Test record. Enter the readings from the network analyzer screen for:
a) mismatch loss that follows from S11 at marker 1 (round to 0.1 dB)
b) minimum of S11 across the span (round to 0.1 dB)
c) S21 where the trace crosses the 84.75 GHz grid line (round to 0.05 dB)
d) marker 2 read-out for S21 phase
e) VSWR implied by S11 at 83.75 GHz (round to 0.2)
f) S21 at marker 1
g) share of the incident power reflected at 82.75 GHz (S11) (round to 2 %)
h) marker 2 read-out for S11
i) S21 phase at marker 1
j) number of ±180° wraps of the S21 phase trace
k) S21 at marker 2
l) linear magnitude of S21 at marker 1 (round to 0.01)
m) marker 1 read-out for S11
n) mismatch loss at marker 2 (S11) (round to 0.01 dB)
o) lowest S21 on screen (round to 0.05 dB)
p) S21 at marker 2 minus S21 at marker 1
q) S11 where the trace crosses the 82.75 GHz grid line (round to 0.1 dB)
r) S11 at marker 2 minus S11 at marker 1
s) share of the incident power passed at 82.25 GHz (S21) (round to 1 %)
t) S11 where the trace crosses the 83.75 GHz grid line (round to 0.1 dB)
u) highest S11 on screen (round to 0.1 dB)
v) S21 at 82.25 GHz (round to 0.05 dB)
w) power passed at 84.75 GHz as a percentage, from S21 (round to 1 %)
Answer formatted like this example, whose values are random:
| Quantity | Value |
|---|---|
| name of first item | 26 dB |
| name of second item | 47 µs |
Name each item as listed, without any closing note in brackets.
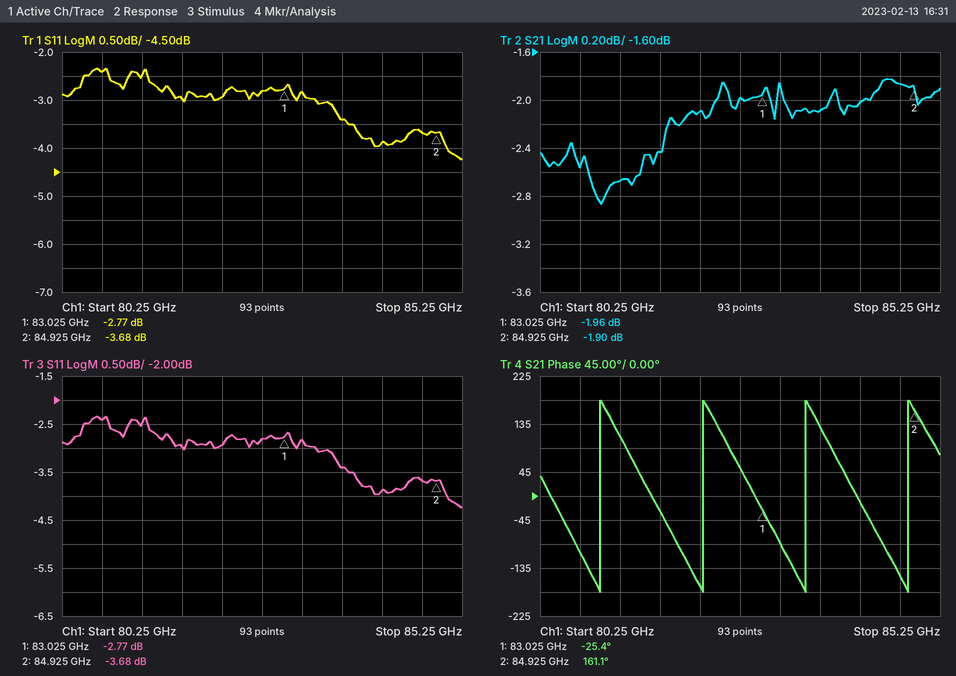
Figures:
| Quantity | Value |
|---|---|
| mismatch loss that follows from S11 at marker 1 | 3.3 dB |
| minimum of S11 across the span | -4.2 dB |
| S21 where the trace crosses the 84.75 GHz grid line | -1.85 dB |
| marker 2 read-out for S21 phase | 161.1° |
| VSWR implied by S11 at 83.75 GHz | 5.2 |
| S21 at marker 1 | -1.96 dB |
| share of the incident power reflected at 82.75 GHz (S11) | 52 % |
| marker 2 read-out for S11 | -3.68 dB |
| S21 phase at marker 1 | -25.4° |
| number of ±180° wraps of the S21 phase trace | 4 |
| S21 at marker 2 | -1.90 dB |
| linear magnitude of S21 at marker 1 | 0.80 |
| marker 1 read-out for S11 | -2.77 dB |
| mismatch loss at marker 2 (S11) | 2.43 dB |
| lowest S21 on screen | -2.85 dB |
| S21 at marker 2 minus S21 at marker 1 | 0.06 dB |
| S11 where the trace crosses the 82.75 GHz grid line | -2.8 dB |
| S11 at marker 2 minus S11 at marker 1 | -0.91 dB |
| share of the incident power passed at 82.25 GHz (S21) | 62 % |
| S11 where the trace crosses the 83.75 GHz grid line | -3.4 dB |
| highest S11 on screen | -2.3 dB |
| S21 at 82.25 GHz | -2.10 dB |
| power passed at 84.75 GHz as a percentage, from S21 | 65 % |
